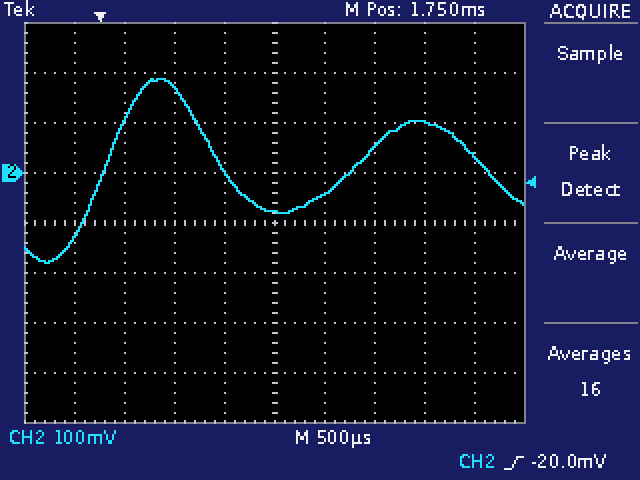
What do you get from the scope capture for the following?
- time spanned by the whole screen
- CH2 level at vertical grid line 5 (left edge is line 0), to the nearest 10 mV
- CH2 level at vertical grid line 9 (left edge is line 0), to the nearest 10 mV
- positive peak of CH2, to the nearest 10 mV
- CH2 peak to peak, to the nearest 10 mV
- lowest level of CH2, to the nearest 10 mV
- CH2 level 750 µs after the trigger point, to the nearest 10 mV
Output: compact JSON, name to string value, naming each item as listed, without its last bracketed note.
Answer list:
{"time spanned by the whole screen": "5 ms", "CH2 level at vertical grid line 5 (left edge is line 0), to the nearest 10 mV": "-80 mV", "CH2 level at vertical grid line 9 (left edge is line 0), to the nearest 10 mV": "30 mV", "positive peak of CH2, to the nearest 10 mV": "190 mV", "CH2 peak to peak, to the nearest 10 mV": "370 mV", "lowest level of CH2, to the nearest 10 mV": "-180 mV", "CH2 level 750 µs after the trigger point, to the nearest 10 mV": "170 mV"}
